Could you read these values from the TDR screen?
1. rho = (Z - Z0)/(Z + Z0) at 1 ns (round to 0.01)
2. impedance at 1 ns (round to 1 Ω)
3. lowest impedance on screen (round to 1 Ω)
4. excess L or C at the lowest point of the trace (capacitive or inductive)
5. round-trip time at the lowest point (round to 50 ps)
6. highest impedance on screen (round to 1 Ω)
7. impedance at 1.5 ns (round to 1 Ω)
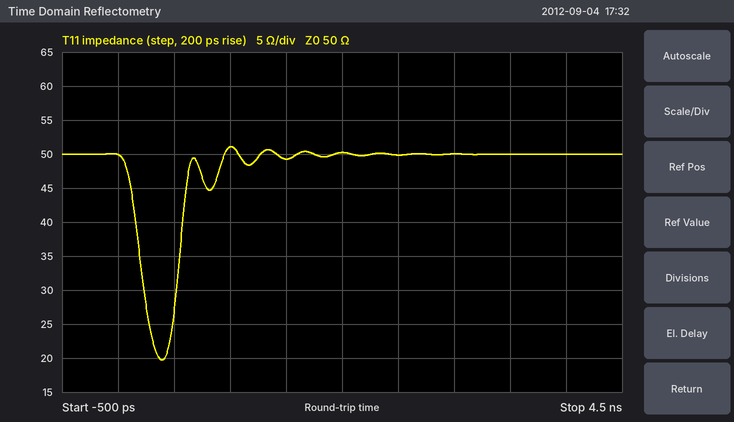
+0.01
51 Ω
20 Ω
capacitive
400 ps
51 Ω
49 Ω
